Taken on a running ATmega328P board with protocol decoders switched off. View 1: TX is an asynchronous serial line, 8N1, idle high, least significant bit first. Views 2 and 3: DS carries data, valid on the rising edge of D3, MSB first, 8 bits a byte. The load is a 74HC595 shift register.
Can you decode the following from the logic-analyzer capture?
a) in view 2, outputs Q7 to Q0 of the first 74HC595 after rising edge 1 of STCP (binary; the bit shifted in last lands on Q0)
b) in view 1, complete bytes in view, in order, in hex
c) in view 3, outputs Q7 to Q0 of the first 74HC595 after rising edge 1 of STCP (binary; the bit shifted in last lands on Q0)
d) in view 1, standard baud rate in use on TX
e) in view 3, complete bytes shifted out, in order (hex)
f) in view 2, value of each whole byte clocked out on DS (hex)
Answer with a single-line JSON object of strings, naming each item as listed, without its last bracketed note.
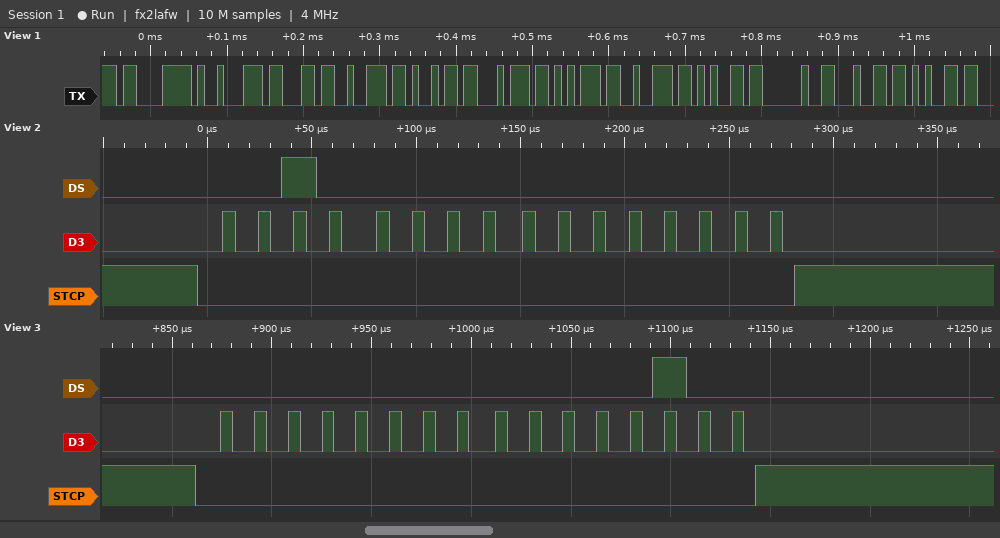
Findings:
{"in view 2, outputs Q7 to Q0 of the first 74HC595 after rising edge 1 of STCP": "00000000", "in view 1, complete bytes in view, in order, in hex": "C3 89 63 72 69 74 75 72 65 20 64 65", "in view 3, outputs Q7 to Q0 of the first 74HC595 after rising edge 1 of STCP": "00000100", "in view 1, standard baud rate in use on TX": "115200 baud", "in view 3, complete bytes shifted out, in order": "00 04", "in view 2, value of each whole byte clocked out on DS": "20 00"}
